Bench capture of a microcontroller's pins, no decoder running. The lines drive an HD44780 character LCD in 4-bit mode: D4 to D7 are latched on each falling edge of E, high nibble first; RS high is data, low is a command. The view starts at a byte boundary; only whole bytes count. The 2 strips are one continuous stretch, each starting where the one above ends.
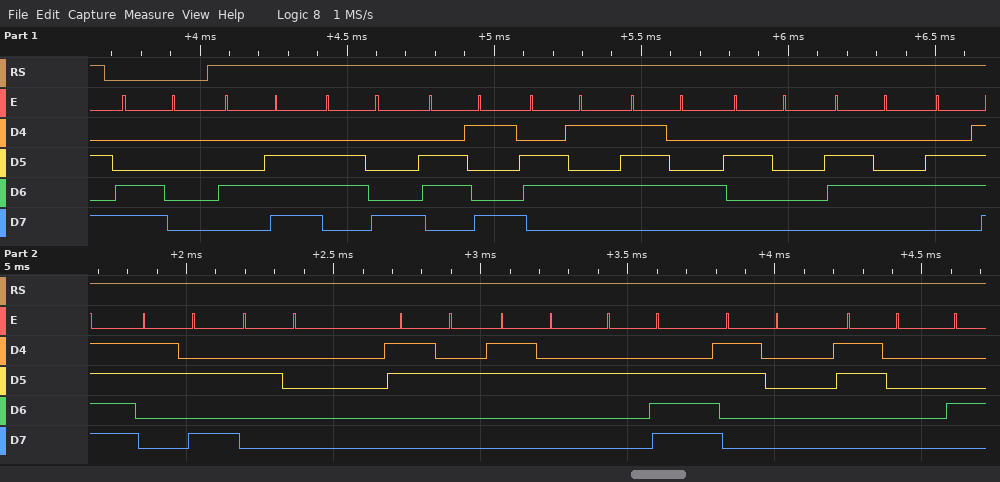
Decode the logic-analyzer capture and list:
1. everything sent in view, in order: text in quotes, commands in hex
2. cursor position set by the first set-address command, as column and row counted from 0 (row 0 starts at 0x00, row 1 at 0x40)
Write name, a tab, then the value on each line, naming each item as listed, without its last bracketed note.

everything sent in view, in order: text in quotes, commands in hex	0xC0 "Nhiet do: 22.00"
cursor position set by the first set-address command, as column and row counted from 0	column 0, row 1
